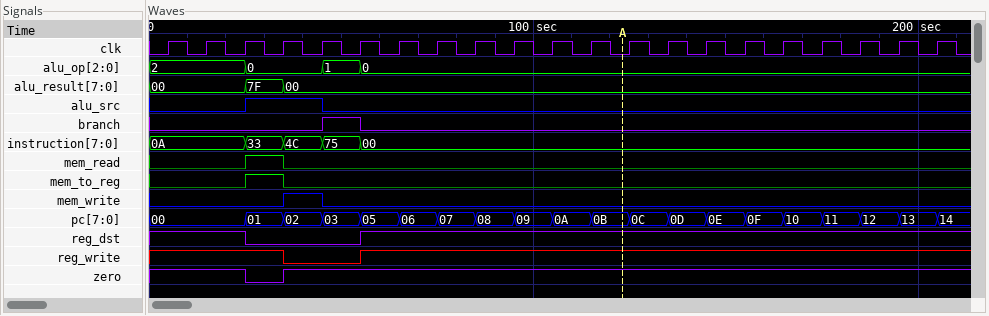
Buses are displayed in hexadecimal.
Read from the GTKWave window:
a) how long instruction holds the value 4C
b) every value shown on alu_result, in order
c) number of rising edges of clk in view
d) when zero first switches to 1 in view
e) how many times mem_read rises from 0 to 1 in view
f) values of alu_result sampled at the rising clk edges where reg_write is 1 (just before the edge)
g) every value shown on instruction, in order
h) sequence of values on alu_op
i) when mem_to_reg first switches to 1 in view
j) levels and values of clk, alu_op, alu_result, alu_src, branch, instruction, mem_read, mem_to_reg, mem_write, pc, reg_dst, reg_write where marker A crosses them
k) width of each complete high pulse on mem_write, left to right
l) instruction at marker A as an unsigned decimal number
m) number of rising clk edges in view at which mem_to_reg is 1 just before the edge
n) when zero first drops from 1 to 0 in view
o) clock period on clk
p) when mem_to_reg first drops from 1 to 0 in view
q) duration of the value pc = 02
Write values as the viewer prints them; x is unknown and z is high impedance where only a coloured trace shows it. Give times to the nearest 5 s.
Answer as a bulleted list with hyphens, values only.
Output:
- 10 s
- 00, 7F, 00
- 21
- 35 s
- 1
- 00, 00, 00, 7F, 00, 00, 00, 00, 00, 00, 00, 00, 00, 00, 00, 00, 00, 00, 00
- 0A, 33, 4C, 75, 00
- 2, 0, 1, 0
- 25 s
- clk=0, alu_op=0, alu_result=00, alu_src=0, branch=0, instruction=00, mem_read=0, mem_to_reg=0, mem_write=0, pc=0B, reg_dst=1, reg_write=1
- 10 s
- 0
- 1
- 25 s
- 10 s
- 35 s
- 10 s
